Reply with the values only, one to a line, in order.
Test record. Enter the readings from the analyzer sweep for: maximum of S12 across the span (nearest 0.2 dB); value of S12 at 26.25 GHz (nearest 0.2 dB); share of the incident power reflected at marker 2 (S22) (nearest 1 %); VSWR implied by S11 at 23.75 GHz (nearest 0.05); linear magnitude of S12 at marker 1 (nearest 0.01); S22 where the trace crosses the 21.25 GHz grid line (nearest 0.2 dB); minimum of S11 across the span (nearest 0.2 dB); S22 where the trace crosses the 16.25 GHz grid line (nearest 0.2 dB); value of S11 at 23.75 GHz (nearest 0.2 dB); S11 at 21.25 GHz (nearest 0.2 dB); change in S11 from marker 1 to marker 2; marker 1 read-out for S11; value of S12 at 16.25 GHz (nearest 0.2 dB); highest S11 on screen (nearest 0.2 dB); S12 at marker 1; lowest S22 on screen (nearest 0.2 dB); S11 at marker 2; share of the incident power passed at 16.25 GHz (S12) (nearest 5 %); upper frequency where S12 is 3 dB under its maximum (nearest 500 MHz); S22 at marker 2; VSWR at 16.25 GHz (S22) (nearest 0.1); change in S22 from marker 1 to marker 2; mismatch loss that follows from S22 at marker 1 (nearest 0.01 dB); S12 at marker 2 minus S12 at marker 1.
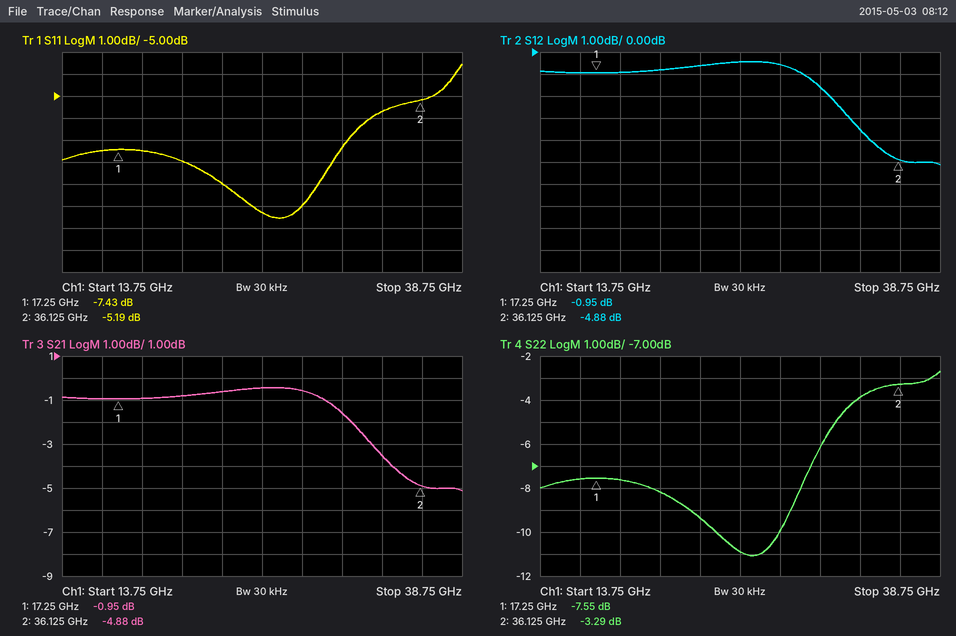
-0.4 dB
-0.4 dB
47 %
2.10
0.90
-8.2 dB
-10.6 dB
-7.6 dB
-9.0 dB
-8.0 dB
2.24 dB
-7.43 dB
-1.0 dB
-3.6 dB
-0.95 dB
-11.0 dB
-5.19 dB
80 %
33.5 GHz
-3.29 dB
2.4
4.26 dB
0.84 dB
-3.93 dB
